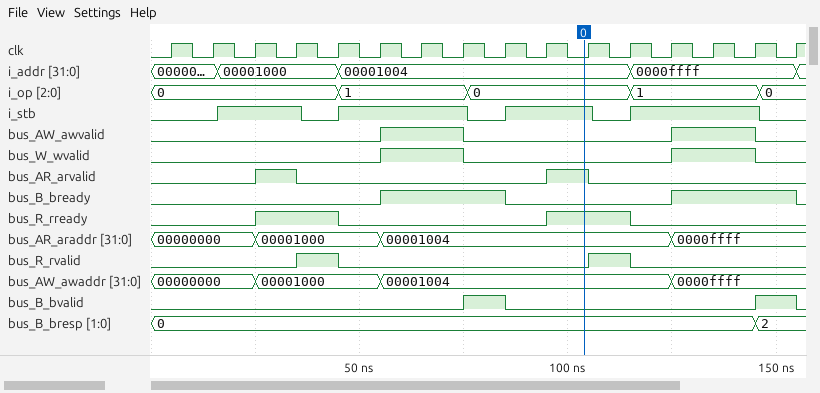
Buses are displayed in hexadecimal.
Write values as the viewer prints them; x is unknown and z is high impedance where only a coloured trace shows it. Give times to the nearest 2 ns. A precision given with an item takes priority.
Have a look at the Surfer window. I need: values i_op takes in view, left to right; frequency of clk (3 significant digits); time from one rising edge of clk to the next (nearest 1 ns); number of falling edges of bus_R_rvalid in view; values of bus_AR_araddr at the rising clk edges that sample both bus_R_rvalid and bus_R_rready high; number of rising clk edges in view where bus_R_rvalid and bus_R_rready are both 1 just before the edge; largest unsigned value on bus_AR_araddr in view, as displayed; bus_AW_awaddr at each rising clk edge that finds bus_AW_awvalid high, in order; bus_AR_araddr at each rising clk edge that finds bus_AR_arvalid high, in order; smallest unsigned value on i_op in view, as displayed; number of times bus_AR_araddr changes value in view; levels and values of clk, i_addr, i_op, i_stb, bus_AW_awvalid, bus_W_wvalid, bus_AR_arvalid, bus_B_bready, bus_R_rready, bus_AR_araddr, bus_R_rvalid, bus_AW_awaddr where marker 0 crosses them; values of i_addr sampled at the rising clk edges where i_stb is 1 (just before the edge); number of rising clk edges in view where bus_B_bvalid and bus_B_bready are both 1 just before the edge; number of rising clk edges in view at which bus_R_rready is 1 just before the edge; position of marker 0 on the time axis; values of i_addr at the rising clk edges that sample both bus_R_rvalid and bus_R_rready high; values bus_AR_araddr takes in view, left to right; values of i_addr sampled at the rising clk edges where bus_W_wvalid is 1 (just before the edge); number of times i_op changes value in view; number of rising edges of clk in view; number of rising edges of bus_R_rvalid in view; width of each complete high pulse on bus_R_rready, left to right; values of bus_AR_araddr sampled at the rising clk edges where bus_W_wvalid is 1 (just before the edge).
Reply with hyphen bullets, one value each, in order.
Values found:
- 0, 1, 0, 1, 0
- 100 MHz
- 10 ns
- 2
- 00001000, 00001004
- 2
- 0000ffff
- 00001004, 00001004, 0000ffff, 0000ffff
- 00001000, 00001004
- 0
- 3
- clk=0, i_addr=00001004, i_op=0, i_stb=1, bus_AW_awvalid=0, bus_W_wvalid=0, bus_AR_arvalid=1, bus_B_bready=0, bus_R_rready=1, bus_AR_araddr=00001004, bus_R_rvalid=0, bus_AW_awaddr=00001004
- 00001000, 00001000, 00001004, 00001004, 00001004, 00001004, 00001004, 0000ffff, 0000ffff, 0000ffff
- 2
- 4
- 104 ns
- 00001000, 00001004
- 00000000, 00001000, 00001004, 0000ffff
- 00001004, 00001004, 0000ffff, 0000ffff
- 4
- 16
- 2
- 20 ns, 20 ns
- 00001004, 00001004, 0000ffff, 0000ffff
